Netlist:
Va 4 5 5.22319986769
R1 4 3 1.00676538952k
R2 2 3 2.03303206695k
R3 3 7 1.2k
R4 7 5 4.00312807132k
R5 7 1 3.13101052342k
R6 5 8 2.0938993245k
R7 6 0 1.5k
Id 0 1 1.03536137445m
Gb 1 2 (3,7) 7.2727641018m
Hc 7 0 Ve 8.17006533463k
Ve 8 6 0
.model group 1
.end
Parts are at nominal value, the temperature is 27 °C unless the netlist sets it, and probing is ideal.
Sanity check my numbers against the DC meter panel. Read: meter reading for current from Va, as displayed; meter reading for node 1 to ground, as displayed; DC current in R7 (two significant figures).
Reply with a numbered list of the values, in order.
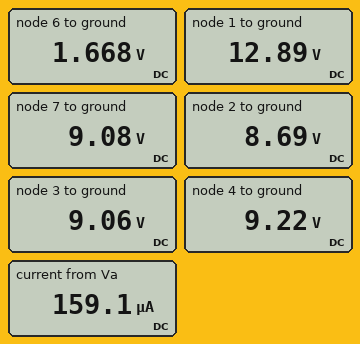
1. 159.1 µA
2. 12.89 V
3. 1.1 mA
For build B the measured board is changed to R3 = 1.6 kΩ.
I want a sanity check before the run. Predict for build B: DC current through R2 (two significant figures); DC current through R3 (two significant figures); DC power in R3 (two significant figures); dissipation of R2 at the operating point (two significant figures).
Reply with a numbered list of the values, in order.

1. 170 µA
2. 15 µA
3. 360 nW
4. 62 µW
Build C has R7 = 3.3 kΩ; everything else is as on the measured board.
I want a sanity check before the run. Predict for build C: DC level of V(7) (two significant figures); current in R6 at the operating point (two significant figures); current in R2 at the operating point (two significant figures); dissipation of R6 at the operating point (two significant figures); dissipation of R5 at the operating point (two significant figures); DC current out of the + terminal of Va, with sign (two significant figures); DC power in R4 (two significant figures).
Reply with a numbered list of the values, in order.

1. 17 V
2. 2.1 mA
3. 720 µA
4. 9.0 mW
5. 310 µW
6. -640 µA
7. 8.3 mW
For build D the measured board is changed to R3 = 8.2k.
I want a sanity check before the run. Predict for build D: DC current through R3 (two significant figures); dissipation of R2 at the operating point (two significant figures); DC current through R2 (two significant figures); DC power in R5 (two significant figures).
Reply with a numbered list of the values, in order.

1. 2.7 µA
2. 53 µW
3. 160 µA
4. 4.5 mW
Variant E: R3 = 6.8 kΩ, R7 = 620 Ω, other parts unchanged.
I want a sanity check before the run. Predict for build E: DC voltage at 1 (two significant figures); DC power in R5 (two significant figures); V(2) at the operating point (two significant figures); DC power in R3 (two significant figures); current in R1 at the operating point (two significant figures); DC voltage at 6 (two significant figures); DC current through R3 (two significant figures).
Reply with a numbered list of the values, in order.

1. 12 V
2. 5.9 mW
3. 6.7 V
4. 310 nW
5. 330 µA
6. 560 mV
7. 6.8 µA
